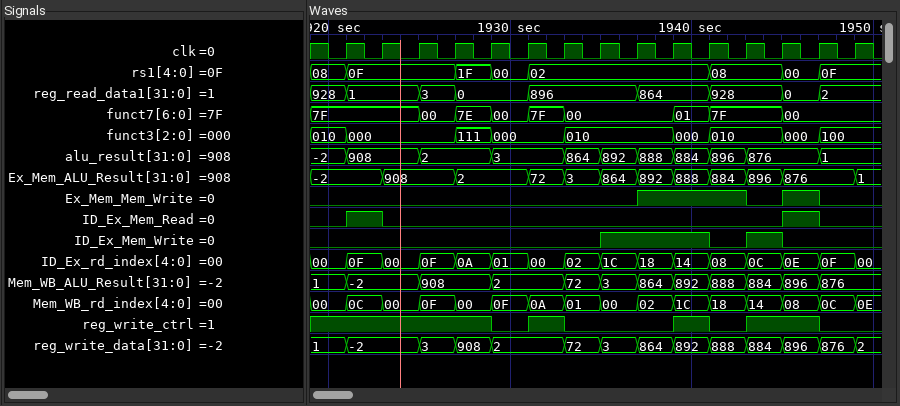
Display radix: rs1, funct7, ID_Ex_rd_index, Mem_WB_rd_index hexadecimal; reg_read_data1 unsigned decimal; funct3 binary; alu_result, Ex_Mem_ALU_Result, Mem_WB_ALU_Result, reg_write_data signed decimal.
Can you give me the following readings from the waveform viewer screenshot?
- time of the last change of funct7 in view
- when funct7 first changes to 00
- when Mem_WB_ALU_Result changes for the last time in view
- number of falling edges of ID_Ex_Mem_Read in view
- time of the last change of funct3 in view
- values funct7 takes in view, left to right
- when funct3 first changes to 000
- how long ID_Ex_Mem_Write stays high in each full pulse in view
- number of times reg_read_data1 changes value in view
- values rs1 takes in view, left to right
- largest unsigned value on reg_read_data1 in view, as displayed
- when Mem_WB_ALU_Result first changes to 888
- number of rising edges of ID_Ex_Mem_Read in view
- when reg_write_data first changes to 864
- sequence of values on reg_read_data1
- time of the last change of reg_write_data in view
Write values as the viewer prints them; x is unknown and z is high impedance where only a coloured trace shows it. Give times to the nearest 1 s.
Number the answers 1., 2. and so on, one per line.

1. 1945 s
2. 1925 s
3. 1947 s
4. 2
5. 1947 s
6. 7F, 00, 7E, 00, 7F, 00, 01, 7F, 00
7. 1921 s
8. 6 s, 2 s
9. 8
10. 08, 0F, 1F, 00, 02, 08, 00, 0F
11. 928
12. 1941 s
13. 2
14. 1937 s
15. 928, 1, 3, 0, 896, 864, 928, 0, 2
16. 1949 s
